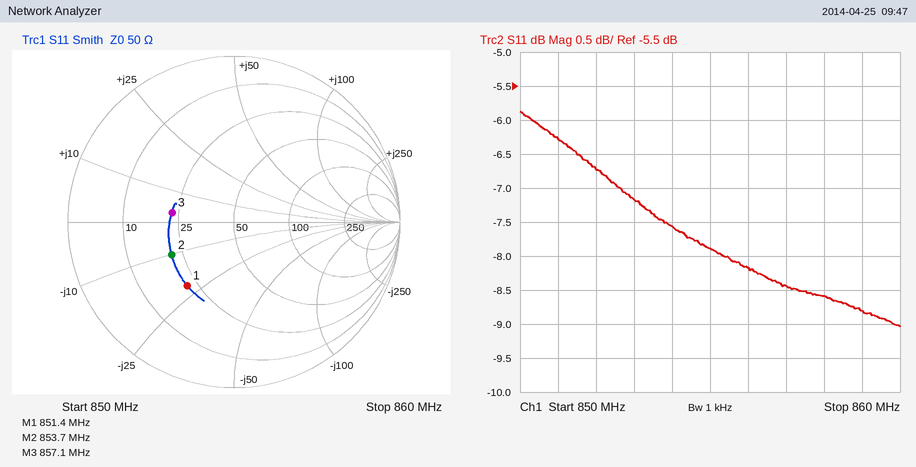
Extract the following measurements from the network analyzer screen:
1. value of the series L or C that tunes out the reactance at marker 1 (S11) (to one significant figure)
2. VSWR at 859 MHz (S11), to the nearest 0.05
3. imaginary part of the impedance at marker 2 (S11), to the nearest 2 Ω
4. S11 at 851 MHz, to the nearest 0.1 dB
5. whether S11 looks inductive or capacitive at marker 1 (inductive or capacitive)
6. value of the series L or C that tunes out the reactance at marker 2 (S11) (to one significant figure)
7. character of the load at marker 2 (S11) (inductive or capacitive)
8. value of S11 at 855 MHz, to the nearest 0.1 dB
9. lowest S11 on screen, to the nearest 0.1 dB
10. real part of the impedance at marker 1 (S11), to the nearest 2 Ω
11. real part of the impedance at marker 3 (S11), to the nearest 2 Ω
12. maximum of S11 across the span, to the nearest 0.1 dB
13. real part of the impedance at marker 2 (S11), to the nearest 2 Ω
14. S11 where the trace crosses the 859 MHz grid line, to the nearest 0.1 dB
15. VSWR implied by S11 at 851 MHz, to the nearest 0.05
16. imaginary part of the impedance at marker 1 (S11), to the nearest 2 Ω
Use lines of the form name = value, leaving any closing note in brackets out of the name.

value of the series L or C that tunes out the reactance at marker 1 (S11) = 4 nH
VSWR at 859 MHz (S11), to the nearest 0.05 = 2.15
imaginary part of the impedance at marker 2 (S11), to the nearest 2 Ω = -10 Ω
S11 at 851 MHz, to the nearest 0.1 dB = -6.3 dB
whether S11 looks inductive or capacitive at marker 1 = capacitive
value of the series L or C that tunes out the reactance at marker 2 (S11) = 2 nH
character of the load at marker 2 (S11) = capacitive
value of S11 at 855 MHz, to the nearest 0.1 dB = -7.9 dB
lowest S11 on screen, to the nearest 0.1 dB = -9.0 dB
real part of the impedance at marker 1 (S11), to the nearest 2 Ω = 22 Ω
real part of the impedance at marker 3 (S11), to the nearest 2 Ω = 22 Ω
maximum of S11 across the span, to the nearest 0.1 dB = -5.9 dB
real part of the impedance at marker 2 (S11), to the nearest 2 Ω = 22 Ω
S11 where the trace crosses the 859 MHz grid line, to the nearest 0.1 dB = -8.8 dB
VSWR implied by S11 at 851 MHz, to the nearest 0.05 = 2.90
imaginary part of the impedance at marker 1 (S11), to the nearest 2 Ω = -22 Ω
